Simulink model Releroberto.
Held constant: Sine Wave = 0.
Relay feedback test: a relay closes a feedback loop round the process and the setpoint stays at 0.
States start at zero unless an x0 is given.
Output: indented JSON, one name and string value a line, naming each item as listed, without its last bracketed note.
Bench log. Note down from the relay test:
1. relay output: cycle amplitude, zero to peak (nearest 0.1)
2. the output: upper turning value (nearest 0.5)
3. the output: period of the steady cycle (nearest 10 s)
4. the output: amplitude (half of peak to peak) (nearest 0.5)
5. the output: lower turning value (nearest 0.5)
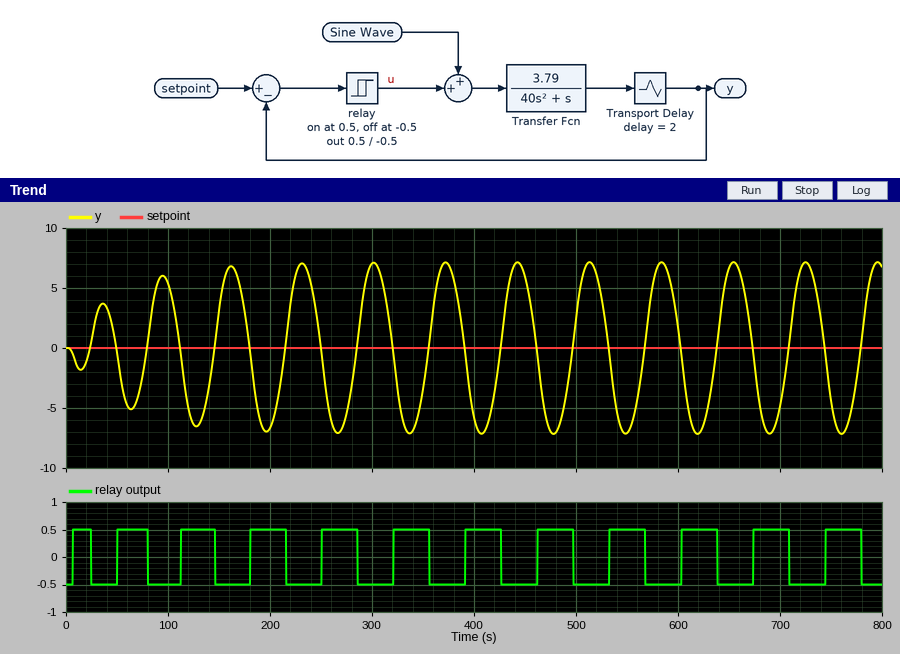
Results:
{
  "relay output: cycle amplitude, zero to peak": "0.5",
  "the output: upper turning value": "7.0",
  "the output: period of the steady cycle": "70 s",
  "the output: amplitude (half of peak to peak)": "7.0",
  "the output: lower turning value": "-7.0"
}
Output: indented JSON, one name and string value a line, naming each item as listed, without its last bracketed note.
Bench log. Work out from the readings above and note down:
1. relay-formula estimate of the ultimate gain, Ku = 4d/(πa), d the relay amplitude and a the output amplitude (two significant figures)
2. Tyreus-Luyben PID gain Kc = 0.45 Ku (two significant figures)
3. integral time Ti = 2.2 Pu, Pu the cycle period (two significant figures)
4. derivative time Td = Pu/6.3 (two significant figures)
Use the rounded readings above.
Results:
{
  "relay-formula estimate of the ultimate gain, Ku = 4d/(πa), d the relay amplitude and a the output amplitude": "0.091",
  "Tyreus-Luyben PID gain Kc = 0.45 Ku": "0.041",
  "integral time Ti = 2.2 Pu, Pu the cycle period": "150 s",
  "derivative time Td = Pu/6.3": "11 s"
}
